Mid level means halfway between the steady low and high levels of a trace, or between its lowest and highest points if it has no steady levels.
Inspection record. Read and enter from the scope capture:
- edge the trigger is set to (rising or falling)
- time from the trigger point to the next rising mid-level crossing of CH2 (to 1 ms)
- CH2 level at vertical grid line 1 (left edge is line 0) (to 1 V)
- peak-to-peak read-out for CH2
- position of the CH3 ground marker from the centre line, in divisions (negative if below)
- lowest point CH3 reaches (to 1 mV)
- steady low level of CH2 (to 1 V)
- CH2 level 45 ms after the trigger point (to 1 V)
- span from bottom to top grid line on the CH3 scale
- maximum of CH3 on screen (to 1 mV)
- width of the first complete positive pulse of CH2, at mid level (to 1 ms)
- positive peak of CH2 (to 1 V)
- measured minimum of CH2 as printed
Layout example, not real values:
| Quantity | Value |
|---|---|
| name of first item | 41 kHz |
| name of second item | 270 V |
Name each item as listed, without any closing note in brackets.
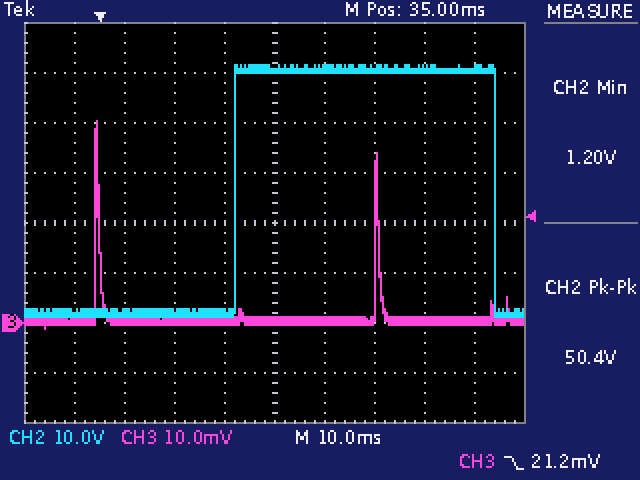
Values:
| Quantity | Value |
|---|---|
| edge the trigger is set to | falling |
| time from the trigger point to the next rising mid-level crossing of CH2 | 27 ms |
| CH2 level at vertical grid line 1 (left edge is line 0) | 2 V |
| peak-to-peak read-out for CH2 | 50.4 V |
| position of the CH3 ground marker from the centre line, in divisions | -2.0 div |
| lowest point CH3 reaches | -1 mV |
| steady low level of CH2 | 2 V |
| CH2 level 45 ms after the trigger point | 51 V |
| span from bottom to top grid line on the CH3 scale | 80 mV |
| maximum of CH3 on screen | 40 mV |
| width of the first complete positive pulse of CH2, at mid level | 52 ms |
| positive peak of CH2 | 52 V |
| measured minimum of CH2 as printed | 1.20 V |
